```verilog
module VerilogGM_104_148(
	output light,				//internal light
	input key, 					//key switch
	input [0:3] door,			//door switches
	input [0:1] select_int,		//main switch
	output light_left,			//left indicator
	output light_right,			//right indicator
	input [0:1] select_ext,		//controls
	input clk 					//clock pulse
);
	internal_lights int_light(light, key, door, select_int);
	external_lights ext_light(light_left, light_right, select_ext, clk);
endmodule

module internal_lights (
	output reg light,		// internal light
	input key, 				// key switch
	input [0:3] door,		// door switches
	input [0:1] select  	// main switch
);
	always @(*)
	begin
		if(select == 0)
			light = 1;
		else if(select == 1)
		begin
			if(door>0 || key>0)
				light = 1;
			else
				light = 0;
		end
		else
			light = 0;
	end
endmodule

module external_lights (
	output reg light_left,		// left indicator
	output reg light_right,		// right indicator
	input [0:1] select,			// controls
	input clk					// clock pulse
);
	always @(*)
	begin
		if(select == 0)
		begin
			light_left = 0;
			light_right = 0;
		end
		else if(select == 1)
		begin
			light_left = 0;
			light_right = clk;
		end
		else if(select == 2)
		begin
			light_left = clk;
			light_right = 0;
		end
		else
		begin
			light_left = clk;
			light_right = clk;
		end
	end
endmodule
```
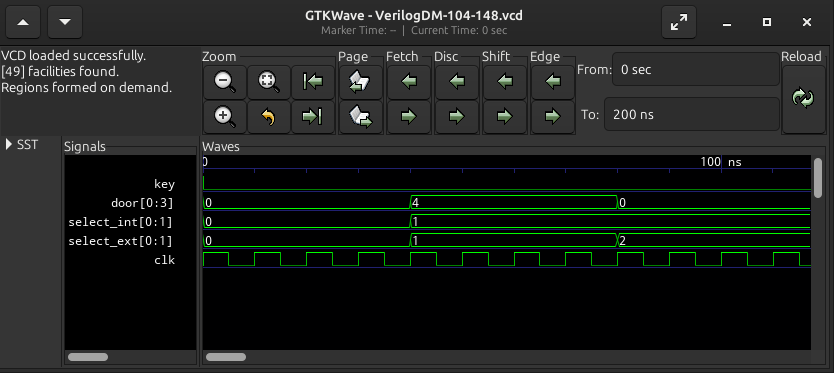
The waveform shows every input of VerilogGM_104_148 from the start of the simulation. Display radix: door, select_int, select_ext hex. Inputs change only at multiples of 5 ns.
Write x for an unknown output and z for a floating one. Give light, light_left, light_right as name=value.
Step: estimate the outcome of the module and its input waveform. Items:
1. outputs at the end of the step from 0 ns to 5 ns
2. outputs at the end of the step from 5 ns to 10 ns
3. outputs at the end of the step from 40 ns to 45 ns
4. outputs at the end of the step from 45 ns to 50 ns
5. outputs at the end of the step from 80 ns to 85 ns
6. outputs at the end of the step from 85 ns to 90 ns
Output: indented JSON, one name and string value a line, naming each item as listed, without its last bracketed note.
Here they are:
{
  "outputs at the end of the step from 0 ns to 5 ns": "light=1, light_left=0, light_right=0",
  "outputs at the end of the step from 5 ns to 10 ns": "light=1, light_left=0, light_right=0",
  "outputs at the end of the step from 40 ns to 45 ns": "light=1, light_left=0, light_right=1",
  "outputs at the end of the step from 45 ns to 50 ns": "light=1, light_left=0, light_right=0",
  "outputs at the end of the step from 80 ns to 85 ns": "light=0, light_left=1, light_right=0",
  "outputs at the end of the step from 85 ns to 90 ns": "light=0, light_left=0, light_right=0"
}
